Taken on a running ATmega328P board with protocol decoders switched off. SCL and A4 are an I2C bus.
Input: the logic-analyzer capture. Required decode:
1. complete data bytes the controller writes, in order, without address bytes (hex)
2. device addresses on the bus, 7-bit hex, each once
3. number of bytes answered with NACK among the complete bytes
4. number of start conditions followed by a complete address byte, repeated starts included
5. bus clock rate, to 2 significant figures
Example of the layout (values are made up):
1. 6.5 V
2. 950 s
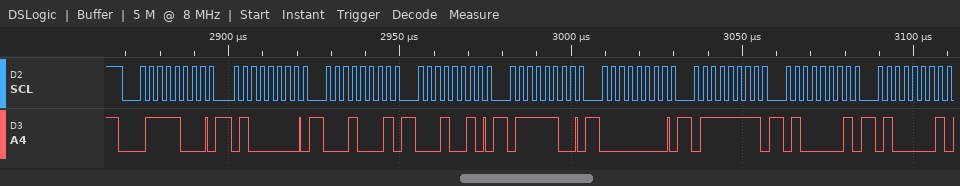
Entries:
1. 40 11 12 7C 00 7F 41 41
2. 0x3C
3. 0
4. 1
5. 400 kHz
